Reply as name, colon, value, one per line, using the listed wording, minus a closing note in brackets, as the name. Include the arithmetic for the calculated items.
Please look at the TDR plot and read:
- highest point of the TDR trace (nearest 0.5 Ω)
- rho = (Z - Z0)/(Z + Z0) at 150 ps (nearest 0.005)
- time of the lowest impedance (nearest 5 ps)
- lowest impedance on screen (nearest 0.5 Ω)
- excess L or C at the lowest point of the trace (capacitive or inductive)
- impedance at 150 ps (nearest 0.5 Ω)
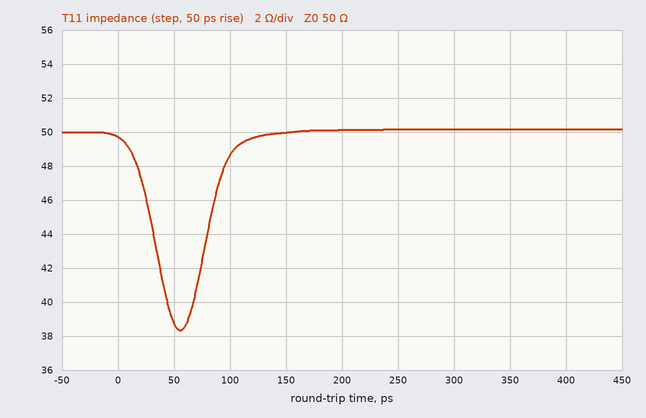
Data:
highest point of the TDR trace: 50.0 Ω
rho = (Z - Z0)/(Z + Z0) at 150 ps: (50 − 50)/(50 + 50) ≈ 0.000
time of the lowest impedance: 55 ps
lowest impedance on screen: 38.5 Ω
excess L or C at the lowest point of the trace: capacitive
impedance at 150 ps: 50.0 Ω
